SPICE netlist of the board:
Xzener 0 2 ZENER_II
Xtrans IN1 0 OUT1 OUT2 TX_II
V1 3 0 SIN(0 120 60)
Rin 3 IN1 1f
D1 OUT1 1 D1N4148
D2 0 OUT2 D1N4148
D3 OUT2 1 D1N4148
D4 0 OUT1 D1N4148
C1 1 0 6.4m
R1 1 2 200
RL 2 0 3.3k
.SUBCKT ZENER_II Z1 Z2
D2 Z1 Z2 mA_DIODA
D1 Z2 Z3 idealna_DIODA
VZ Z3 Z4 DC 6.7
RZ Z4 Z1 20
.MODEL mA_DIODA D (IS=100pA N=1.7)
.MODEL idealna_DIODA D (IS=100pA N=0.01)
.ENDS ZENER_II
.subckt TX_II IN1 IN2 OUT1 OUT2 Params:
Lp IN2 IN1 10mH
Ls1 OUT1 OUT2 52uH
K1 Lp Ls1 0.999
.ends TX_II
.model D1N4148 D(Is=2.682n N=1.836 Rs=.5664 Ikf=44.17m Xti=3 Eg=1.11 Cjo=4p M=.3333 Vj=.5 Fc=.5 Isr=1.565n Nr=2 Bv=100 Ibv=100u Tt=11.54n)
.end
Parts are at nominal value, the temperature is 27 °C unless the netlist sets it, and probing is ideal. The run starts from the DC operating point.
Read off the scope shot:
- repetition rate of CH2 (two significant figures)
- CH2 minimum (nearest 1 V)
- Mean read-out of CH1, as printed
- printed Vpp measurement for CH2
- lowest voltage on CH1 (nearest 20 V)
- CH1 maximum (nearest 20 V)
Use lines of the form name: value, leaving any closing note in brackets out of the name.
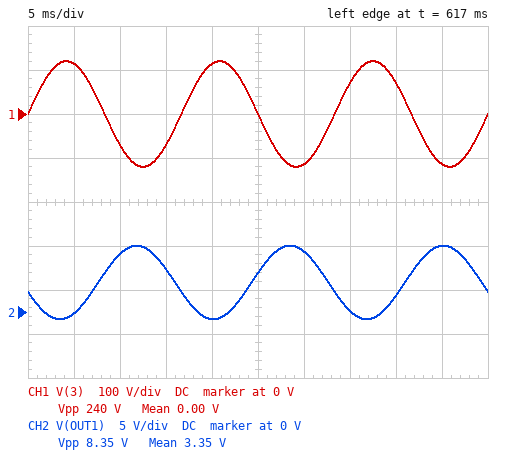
repetition rate of CH2: 60 Hz
CH2 minimum: -1 V
Mean read-out of CH1, as printed: 0.00 V
printed Vpp measurement for CH2: 8.35 V
lowest voltage on CH1: -120 V
CH1 maximum: 120 V
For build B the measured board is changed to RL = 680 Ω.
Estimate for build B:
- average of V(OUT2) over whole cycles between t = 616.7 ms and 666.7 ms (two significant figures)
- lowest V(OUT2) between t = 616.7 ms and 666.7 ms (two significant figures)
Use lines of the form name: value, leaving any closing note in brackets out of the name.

average of V(OUT2) over whole cycles between t = 616.7 ms and 666.7 ms: 3.3 V
lowest V(OUT2) between t = 616.7 ms and 666.7 ms: -900 mV
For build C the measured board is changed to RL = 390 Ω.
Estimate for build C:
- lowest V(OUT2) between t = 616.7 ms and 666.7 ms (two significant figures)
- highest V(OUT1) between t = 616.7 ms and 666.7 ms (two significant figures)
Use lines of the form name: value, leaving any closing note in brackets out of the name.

lowest V(OUT2) between t = 616.7 ms and 666.7 ms: -930 mV
highest V(OUT1) between t = 616.7 ms and 666.7 ms: 7.4 V
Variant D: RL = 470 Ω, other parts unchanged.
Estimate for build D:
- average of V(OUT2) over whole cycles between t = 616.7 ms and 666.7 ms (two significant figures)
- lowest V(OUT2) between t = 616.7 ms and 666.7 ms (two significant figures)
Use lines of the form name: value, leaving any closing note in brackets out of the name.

average of V(OUT2) over whole cycles between t = 616.7 ms and 666.7 ms: 3.3 V
lowest V(OUT2) between t = 616.7 ms and 666.7 ms: -920 mV
